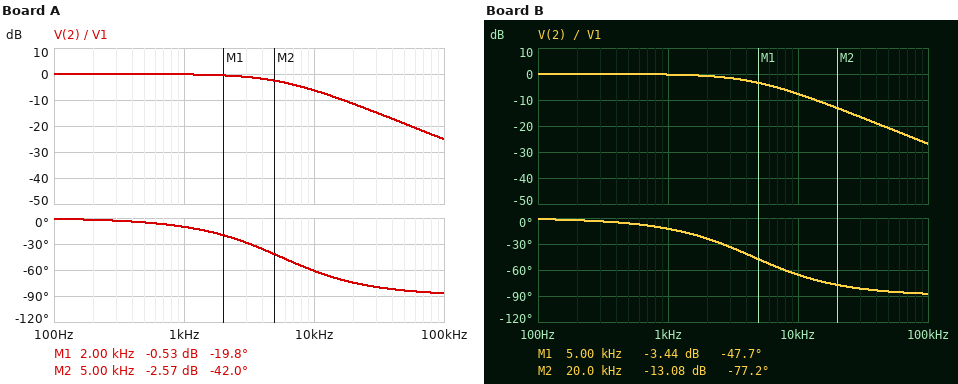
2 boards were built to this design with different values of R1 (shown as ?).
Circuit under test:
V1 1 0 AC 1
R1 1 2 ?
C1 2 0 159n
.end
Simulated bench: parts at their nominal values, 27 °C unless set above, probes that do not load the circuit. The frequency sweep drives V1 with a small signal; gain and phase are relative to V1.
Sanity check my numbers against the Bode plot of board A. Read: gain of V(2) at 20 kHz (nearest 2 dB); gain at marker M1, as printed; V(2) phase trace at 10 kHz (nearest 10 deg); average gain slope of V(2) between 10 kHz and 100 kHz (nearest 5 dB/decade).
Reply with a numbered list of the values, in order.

1. -12 dB
2. -0.53 dB
3. -60 deg
4. -20 dB/decade
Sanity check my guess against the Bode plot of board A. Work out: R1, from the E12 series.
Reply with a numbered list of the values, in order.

1. 180 Ω
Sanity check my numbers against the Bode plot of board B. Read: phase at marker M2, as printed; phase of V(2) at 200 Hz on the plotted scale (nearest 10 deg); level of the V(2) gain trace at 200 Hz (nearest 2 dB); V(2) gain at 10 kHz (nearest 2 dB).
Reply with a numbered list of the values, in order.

1. -77.2 deg
2. 0 deg
3. 0 dB
4. -8 dB
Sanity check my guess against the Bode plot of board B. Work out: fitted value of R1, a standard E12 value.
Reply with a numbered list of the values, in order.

1. 220 Ω
